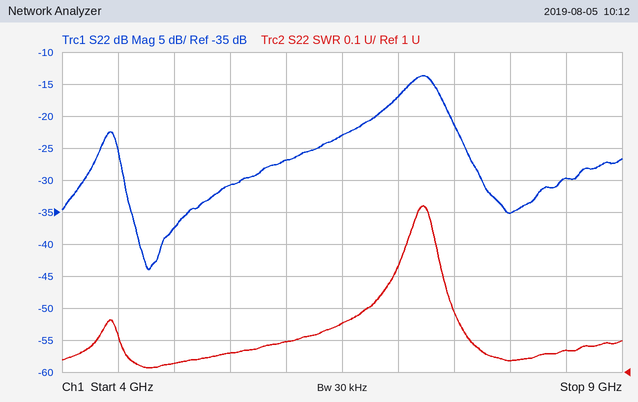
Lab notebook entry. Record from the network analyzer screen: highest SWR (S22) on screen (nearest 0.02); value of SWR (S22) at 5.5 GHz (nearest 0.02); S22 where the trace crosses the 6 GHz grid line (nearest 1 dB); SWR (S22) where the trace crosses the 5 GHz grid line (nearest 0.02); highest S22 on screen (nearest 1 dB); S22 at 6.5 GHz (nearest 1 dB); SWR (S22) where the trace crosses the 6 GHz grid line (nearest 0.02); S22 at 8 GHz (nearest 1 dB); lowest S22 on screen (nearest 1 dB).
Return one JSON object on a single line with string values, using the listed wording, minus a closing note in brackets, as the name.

{"highest SWR (S22) on screen": "1.52", "value of SWR (S22) at 5.5 GHz": "1.06", "S22 where the trace crosses the 6 GHz grid line": "-27 dB", "SWR (S22) where the trace crosses the 5 GHz grid line": "1.02", "highest S22 on screen": "-14 dB", "S22 at 6.5 GHz": "-23 dB", "SWR (S22) where the trace crosses the 6 GHz grid line": "1.10", "S22 at 8 GHz": "-35 dB", "lowest S22 on screen": "-44 dB"}
